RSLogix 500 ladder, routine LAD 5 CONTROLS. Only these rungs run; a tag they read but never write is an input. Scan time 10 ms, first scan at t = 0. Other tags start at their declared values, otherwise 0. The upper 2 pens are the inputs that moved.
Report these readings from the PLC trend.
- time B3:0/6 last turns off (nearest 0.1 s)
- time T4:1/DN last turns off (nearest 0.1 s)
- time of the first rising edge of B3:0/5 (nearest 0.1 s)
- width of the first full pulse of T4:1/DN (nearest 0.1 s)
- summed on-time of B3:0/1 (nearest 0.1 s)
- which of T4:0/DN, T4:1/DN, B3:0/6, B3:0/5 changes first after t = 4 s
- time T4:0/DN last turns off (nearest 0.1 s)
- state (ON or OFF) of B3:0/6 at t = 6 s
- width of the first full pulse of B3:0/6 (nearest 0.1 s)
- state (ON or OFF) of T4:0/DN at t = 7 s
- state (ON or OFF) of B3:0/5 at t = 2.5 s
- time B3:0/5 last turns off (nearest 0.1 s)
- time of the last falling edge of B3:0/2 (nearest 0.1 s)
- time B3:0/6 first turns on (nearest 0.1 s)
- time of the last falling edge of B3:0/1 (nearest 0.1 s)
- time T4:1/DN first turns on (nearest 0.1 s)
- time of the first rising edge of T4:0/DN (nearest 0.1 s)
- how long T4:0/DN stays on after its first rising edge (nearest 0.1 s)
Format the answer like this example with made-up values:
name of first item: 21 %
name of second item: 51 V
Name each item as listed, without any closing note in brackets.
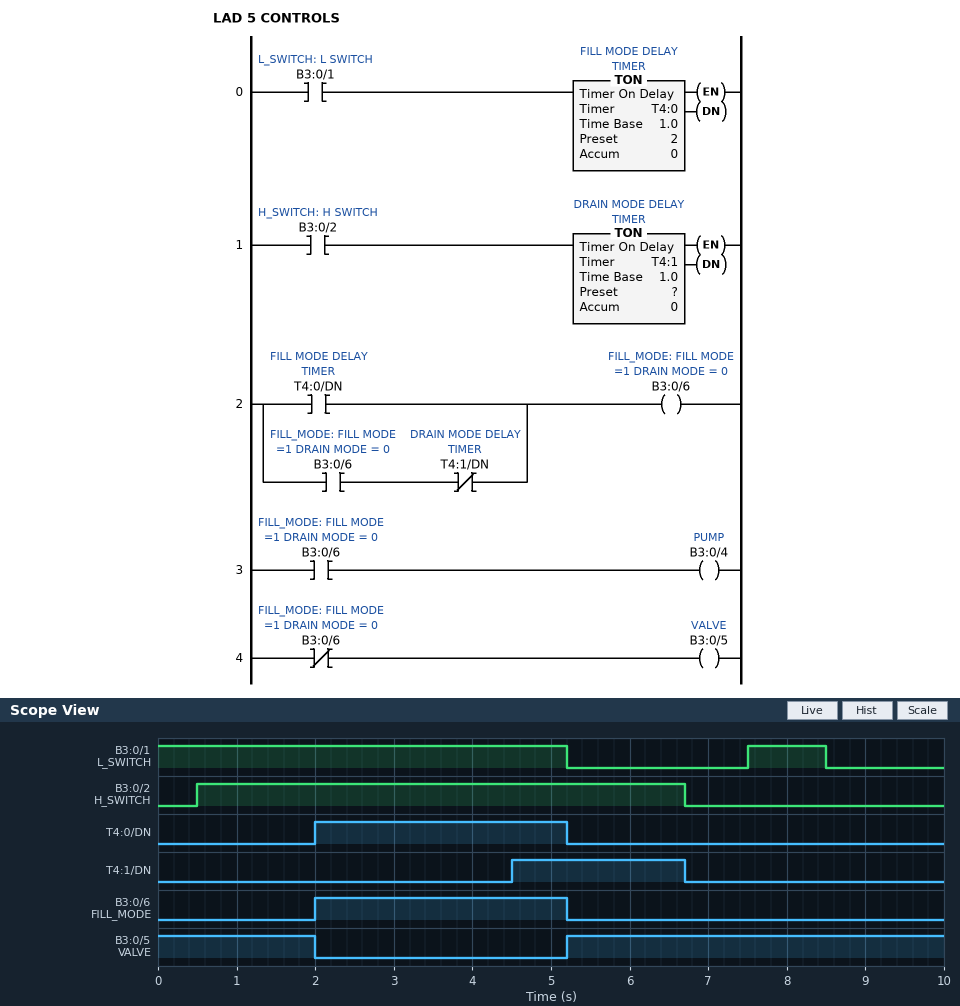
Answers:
time B3:0/6 last turns off: 5.2 s
time T4:1/DN last turns off: 6.7 s
time of the first rising edge of B3:0/5: 5.2 s
width of the first full pulse of T4:1/DN: 2.2 s
summed on-time of B3:0/1: 6.2 s
which of T4:0/DN, T4:1/DN, B3:0/6, B3:0/5 changes first after t = 4 s: T4:1/DN
time T4:0/DN last turns off: 5.2 s
state (ON or OFF) of B3:0/6 at t = 6 s: OFF
width of the first full pulse of B3:0/6: 3.2 s
state (ON or OFF) of T4:0/DN at t = 7 s: OFF
state (ON or OFF) of B3:0/5 at t = 2.5 s: OFF
time B3:0/5 last turns off: 2.0 s
time of the last falling edge of B3:0/2: 6.7 s
time B3:0/6 first turns on: 2.0 s
time of the last falling edge of B3:0/1: 8.5 s
time T4:1/DN first turns on: 4.5 s
time of the first rising edge of T4:0/DN: 2.0 s
how long T4:0/DN stays on after its first rising edge: 3.2 s
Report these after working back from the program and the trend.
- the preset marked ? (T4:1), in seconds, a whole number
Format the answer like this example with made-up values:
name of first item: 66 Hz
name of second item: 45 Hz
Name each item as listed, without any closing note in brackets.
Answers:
the preset marked ? (T4:1), in seconds, a whole number: 4 s
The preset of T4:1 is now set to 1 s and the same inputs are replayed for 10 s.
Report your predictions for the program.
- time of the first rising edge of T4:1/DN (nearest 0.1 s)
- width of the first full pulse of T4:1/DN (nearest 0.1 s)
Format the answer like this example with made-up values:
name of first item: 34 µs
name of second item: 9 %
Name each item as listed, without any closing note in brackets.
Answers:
time of the first rising edge of T4:1/DN: 1.5 s
width of the first full pulse of T4:1/DN: 5.2 s
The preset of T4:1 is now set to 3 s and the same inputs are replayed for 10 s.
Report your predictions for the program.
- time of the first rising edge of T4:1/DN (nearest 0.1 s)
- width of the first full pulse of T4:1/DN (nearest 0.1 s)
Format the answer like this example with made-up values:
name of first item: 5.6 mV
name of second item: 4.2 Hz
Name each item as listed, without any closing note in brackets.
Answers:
time of the first rising edge of T4:1/DN: 3.5 s
width of the first full pulse of T4:1/DN: 3.2 s
